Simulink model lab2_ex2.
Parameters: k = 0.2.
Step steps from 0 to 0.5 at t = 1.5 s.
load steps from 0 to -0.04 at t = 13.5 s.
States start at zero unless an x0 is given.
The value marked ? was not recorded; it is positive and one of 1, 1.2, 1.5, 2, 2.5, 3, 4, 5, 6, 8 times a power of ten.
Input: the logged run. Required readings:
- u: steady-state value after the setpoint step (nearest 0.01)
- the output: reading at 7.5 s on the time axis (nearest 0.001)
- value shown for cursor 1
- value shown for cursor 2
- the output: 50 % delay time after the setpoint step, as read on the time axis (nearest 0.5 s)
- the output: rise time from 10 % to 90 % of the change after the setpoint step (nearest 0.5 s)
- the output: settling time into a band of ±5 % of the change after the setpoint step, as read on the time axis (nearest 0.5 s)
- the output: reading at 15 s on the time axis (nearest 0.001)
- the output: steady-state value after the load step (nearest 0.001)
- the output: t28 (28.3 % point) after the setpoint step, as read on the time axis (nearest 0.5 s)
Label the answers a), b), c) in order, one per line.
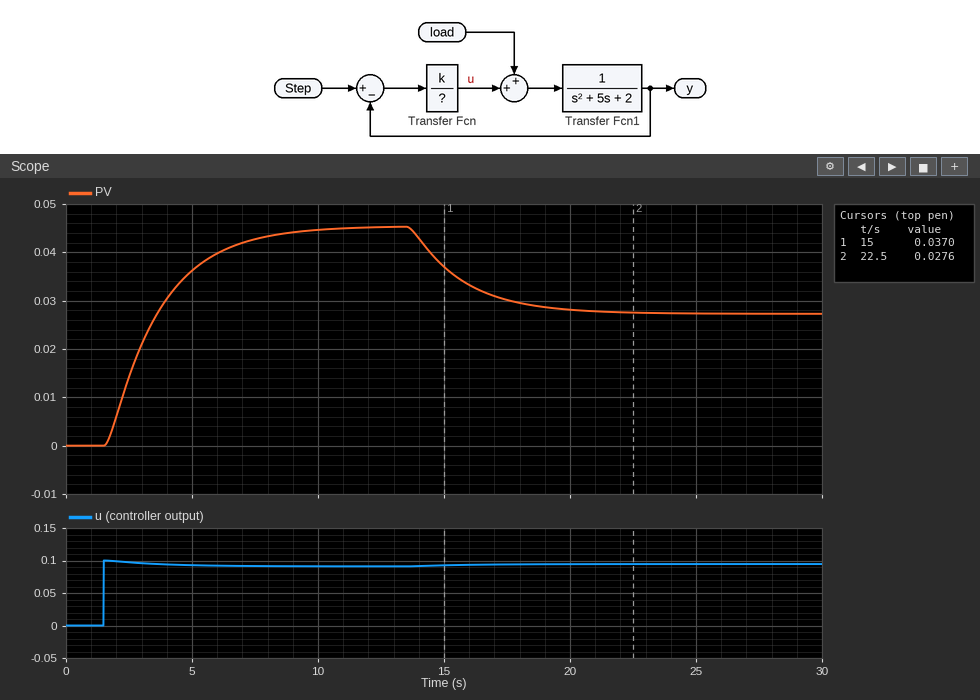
a) 0.09
b) 0.043
c) 0.0370
d) 0.0276
e) 3.0 s
f) 4.5 s
g) 8.0 s
h) 0.037
i) 0.027
j) 2.5 s
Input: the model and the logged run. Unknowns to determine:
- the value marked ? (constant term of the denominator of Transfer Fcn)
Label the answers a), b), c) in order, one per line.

a) 1
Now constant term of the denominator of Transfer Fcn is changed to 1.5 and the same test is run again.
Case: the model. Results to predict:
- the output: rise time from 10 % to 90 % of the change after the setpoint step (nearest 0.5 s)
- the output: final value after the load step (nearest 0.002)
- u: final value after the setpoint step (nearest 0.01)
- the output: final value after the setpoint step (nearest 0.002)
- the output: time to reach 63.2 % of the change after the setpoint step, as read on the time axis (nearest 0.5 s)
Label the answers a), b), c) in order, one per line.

a) 4.5 s
b) 0.012
c) 0.06
d) 0.032
e) 4.0 s
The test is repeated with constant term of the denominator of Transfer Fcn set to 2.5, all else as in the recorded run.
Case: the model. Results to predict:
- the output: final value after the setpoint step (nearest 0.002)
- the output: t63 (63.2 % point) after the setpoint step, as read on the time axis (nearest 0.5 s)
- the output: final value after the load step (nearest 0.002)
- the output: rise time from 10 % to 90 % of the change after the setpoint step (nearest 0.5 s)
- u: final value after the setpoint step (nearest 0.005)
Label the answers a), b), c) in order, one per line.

a) 0.020
b) 4.0 s
c) 0.000
d) 5.0 s
e) 0.040
